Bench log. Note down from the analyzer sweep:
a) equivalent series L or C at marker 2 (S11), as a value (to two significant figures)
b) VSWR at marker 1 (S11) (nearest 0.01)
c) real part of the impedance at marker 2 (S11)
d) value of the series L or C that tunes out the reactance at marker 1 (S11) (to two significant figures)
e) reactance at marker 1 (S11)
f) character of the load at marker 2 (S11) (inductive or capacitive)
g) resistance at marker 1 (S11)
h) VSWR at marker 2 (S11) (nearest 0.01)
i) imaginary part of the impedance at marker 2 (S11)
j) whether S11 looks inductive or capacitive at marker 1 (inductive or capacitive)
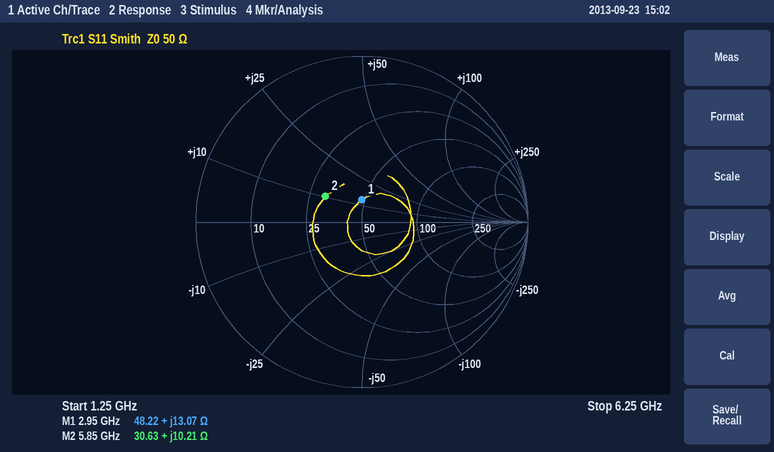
280 pH
1.31
30.63 Ω
4.1 pF
+13.07 Ω
inductive
48.22 Ω
1.74
+10.21 Ω
inductive
